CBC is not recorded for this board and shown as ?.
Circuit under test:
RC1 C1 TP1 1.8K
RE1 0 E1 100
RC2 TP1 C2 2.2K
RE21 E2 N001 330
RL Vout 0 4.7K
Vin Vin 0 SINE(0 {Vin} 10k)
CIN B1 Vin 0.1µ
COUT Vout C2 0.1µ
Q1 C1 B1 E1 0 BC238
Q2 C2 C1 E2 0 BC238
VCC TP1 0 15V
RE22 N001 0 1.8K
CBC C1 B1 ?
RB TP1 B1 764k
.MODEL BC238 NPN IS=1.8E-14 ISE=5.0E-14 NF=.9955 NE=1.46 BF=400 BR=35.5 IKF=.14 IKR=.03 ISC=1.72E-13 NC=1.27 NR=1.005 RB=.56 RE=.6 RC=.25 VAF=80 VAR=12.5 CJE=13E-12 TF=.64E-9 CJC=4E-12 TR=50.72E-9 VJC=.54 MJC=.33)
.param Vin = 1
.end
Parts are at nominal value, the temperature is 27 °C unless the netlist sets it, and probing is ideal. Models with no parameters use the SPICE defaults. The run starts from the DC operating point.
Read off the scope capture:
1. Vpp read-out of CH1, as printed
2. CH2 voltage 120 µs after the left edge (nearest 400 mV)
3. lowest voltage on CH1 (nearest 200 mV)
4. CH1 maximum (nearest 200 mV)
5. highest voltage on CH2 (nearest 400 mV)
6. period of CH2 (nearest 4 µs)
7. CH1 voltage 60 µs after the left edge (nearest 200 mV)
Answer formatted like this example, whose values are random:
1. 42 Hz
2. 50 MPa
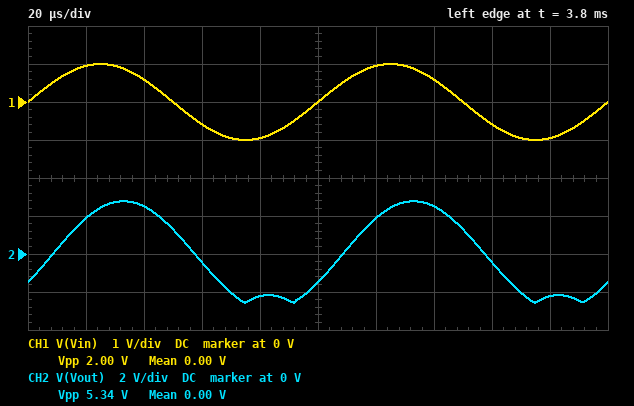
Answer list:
1. 2.00 V
2. 2.0 V
3. -1.0 V
4. 1.0 V
5. 2.8 V
6. 100 µs
7. -600 mV
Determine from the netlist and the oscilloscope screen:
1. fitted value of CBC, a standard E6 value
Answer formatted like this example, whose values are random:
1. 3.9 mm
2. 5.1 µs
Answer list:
1. 15 nF
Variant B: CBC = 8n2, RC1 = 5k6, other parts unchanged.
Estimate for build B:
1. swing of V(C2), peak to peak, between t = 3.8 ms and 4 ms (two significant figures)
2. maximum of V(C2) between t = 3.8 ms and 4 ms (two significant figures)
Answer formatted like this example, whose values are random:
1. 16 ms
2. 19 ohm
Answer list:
1. 5.7 V
2. 14 V
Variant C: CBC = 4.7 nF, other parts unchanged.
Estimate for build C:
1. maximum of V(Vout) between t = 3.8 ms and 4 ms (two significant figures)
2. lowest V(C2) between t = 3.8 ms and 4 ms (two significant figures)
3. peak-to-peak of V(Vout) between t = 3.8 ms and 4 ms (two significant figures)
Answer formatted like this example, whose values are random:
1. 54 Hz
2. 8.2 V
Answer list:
1. 2.9 V
2. 7.9 V
3. 5.5 V
